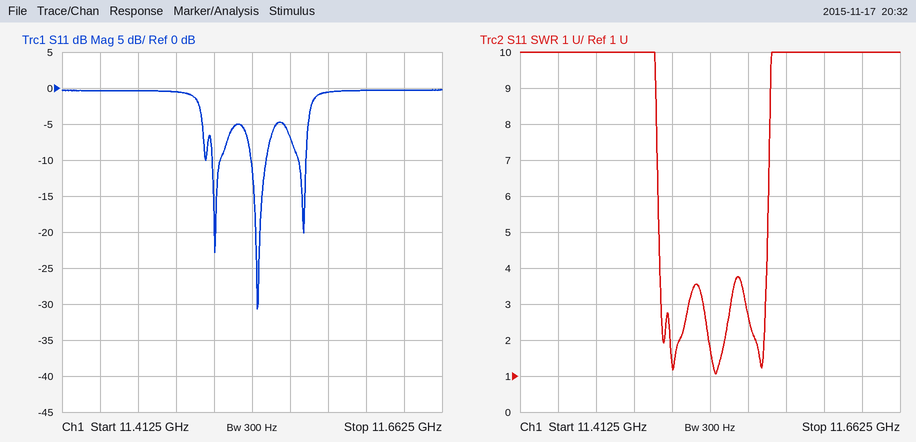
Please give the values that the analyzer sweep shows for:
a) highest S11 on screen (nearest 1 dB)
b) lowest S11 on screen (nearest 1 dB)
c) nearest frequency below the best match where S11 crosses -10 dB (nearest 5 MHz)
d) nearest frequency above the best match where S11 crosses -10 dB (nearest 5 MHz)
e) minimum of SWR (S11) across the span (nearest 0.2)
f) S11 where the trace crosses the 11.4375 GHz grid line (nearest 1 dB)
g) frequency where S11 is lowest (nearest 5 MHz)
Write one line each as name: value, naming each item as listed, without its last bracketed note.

highest S11 on screen: 0 dB
lowest S11 on screen: -31 dB
nearest frequency below the best match where S11 crosses -10 dB: 11.535 GHz
nearest frequency above the best match where S11 crosses -10 dB: 11.545 GHz
minimum of SWR (S11) across the span: 1.0
S11 where the trace crosses the 11.4375 GHz grid line: 0 dB
frequency where S11 is lowest: 11.540 GHz
